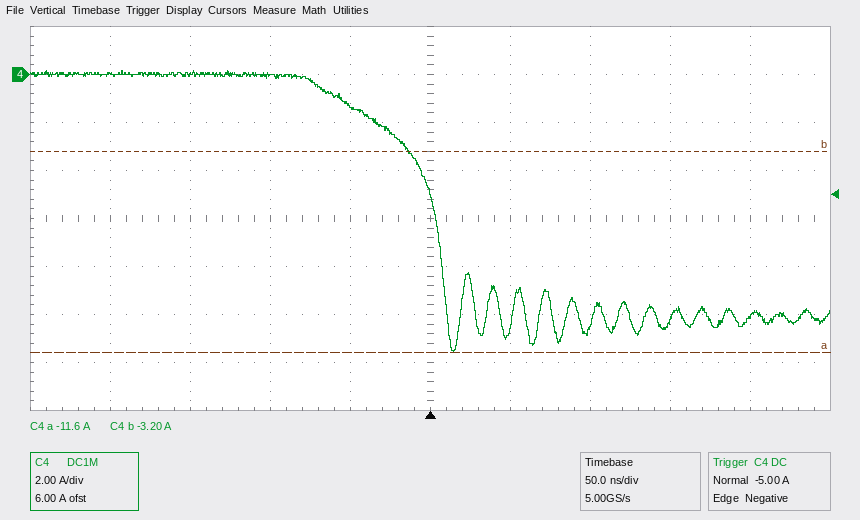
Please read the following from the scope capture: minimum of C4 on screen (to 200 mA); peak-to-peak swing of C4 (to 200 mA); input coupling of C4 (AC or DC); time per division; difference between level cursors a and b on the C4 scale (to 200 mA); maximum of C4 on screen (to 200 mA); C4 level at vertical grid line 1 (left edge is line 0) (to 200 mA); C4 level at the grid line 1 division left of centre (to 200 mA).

-11.6 A
11.8 A
DC
50 ns
8.4 A
200 mA
0.0 A
-1.2 A
